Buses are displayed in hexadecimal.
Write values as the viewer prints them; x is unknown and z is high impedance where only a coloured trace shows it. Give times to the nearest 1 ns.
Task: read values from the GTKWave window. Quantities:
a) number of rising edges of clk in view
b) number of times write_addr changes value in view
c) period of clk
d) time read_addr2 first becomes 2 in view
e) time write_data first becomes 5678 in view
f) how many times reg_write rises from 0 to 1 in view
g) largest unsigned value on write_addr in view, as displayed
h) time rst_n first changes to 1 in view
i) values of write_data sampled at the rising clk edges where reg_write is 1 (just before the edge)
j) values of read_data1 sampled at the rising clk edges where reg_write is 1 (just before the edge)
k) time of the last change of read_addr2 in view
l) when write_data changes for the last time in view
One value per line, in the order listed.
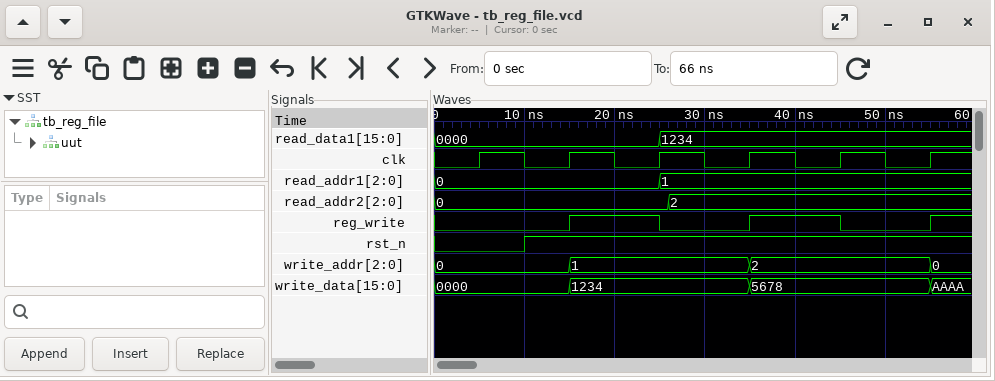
6
3
10 ns
26 ns
35 ns
3
2
10 ns
1234, 5678
0000, 1234
26 ns
55 ns
